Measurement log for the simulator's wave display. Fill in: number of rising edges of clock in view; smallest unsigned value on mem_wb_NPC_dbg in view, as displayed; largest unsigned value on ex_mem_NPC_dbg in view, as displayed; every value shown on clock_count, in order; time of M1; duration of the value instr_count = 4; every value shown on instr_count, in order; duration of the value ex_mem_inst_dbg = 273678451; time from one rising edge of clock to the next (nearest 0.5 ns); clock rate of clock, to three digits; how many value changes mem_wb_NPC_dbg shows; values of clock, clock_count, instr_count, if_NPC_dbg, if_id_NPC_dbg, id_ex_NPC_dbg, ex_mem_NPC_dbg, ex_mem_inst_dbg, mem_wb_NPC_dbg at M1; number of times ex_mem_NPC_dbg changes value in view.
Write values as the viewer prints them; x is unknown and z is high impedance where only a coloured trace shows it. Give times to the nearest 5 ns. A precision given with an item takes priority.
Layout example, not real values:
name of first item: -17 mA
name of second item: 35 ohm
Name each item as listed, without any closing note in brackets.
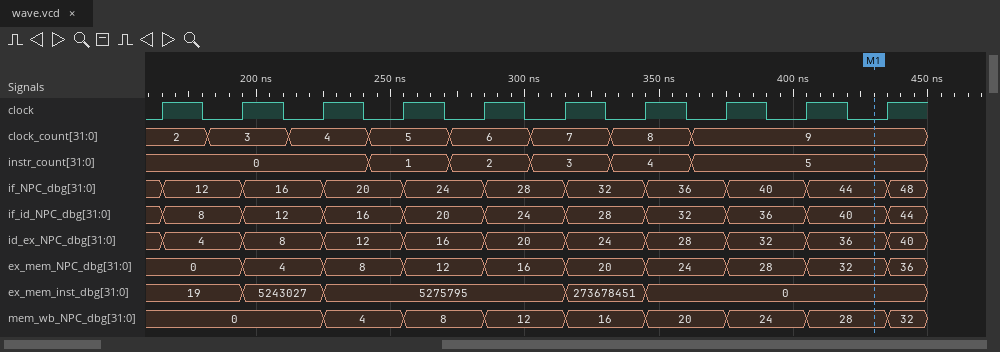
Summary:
number of rising edges of clock in view: 10
smallest unsigned value on mem_wb_NPC_dbg in view, as displayed: 0
largest unsigned value on ex_mem_NPC_dbg in view, as displayed: 36
every value shown on clock_count, in order: 2, 3, 4, 5, 6, 7, 8, 9
time of M1: 430 ns
duration of the value instr_count = 4: 30 ns
every value shown on instr_count, in order: 0, 1, 2, 3, 4, 5
duration of the value ex_mem_inst_dbg = 273678451: 30 ns
time from one rising edge of clock to the next: 30 ns
clock rate of clock, to three digits: 33.3 MHz
how many value changes mem_wb_NPC_dbg shows: 8
values of clock, clock_count, instr_count, if_NPC_dbg, if_id_NPC_dbg, id_ex_NPC_dbg, ex_mem_NPC_dbg, ex_mem_inst_dbg, mem_wb_NPC_dbg at M1: clock=0, clock_count=9, instr_count=5, if_NPC_dbg=44, if_id_NPC_dbg=40, id_ex_NPC_dbg=36, ex_mem_NPC_dbg=32, ex_mem_inst_dbg=0, mem_wb_NPC_dbg=28
number of times ex_mem_NPC_dbg changes value in view: 9
